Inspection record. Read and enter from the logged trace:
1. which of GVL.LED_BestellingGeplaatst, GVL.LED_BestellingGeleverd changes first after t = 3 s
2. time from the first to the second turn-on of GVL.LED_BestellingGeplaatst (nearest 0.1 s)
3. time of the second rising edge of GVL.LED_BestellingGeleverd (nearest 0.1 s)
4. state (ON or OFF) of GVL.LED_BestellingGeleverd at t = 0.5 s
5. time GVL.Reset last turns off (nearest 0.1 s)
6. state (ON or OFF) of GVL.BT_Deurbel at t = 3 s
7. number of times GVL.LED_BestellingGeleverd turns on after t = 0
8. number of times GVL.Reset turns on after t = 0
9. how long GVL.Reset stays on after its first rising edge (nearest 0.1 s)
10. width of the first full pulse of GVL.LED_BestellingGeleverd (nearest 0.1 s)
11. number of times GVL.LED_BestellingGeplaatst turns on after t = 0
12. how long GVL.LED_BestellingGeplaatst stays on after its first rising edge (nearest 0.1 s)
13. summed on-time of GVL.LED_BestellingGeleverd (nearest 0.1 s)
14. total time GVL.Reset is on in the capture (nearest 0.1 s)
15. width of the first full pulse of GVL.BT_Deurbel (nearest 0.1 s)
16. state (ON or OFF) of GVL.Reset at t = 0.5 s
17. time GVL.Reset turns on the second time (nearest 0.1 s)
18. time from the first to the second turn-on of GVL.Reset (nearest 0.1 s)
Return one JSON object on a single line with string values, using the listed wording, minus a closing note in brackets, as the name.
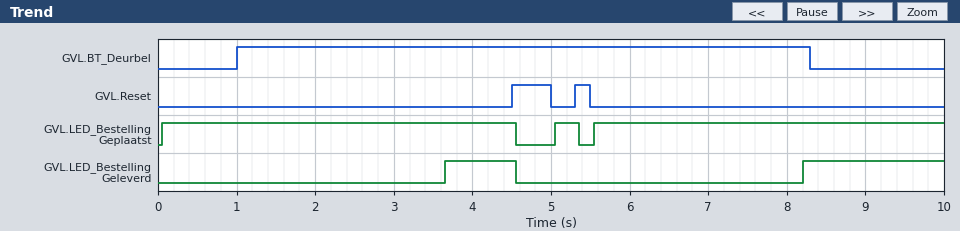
{"which of GVL.LED_BestellingGeplaatst, GVL.LED_BestellingGeleverd changes first after t = 3 s": "GVL.LED_BestellingGeleverd", "time from the first to the second turn-on of GVL.LED_BestellingGeplaatst": "5.0 s", "time of the second rising edge of GVL.LED_BestellingGeleverd": "8.2 s", "state (ON or OFF) of GVL.LED_BestellingGeleverd at t = 0.5 s": "OFF", "time GVL.Reset last turns off": "5.5 s", "state (ON or OFF) of GVL.BT_Deurbel at t = 3 s": "ON", "number of times GVL.LED_BestellingGeleverd turns on after t = 0": "2", "number of times GVL.Reset turns on after t = 0": "2", "how long GVL.Reset stays on after its first rising edge": "0.5 s", "width of the first full pulse of GVL.LED_BestellingGeleverd": "0.9 s", "number of times GVL.LED_BestellingGeplaatst turns on after t = 0": "3", "how long GVL.LED_BestellingGeplaatst stays on after its first rising edge": "4.5 s", "summed on-time of GVL.LED_BestellingGeleverd": "2.7 s", "total time GVL.Reset is on in the capture": "0.7 s", "width of the first full pulse of GVL.BT_Deurbel": "7.3 s", "state (ON or OFF) of GVL.Reset at t = 0.5 s": "OFF", "time GVL.Reset turns on the second time": "5.3 s", "time from the first to the second turn-on of GVL.Reset": "0.8 s"}
